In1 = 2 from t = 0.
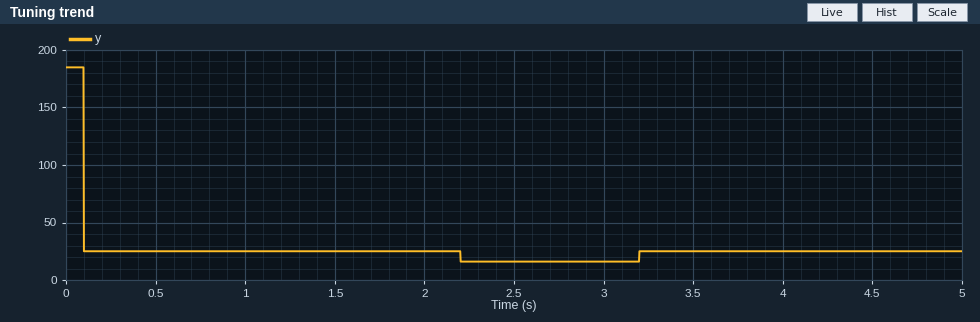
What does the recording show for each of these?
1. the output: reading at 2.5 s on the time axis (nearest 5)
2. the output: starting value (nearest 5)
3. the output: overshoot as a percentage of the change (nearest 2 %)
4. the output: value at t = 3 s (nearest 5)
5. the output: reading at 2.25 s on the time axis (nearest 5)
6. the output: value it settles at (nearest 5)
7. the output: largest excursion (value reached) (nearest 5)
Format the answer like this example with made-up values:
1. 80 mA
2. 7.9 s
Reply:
1. 15
2. 185
3. 6 %
4. 15
5. 15
6. 25
7. 15
